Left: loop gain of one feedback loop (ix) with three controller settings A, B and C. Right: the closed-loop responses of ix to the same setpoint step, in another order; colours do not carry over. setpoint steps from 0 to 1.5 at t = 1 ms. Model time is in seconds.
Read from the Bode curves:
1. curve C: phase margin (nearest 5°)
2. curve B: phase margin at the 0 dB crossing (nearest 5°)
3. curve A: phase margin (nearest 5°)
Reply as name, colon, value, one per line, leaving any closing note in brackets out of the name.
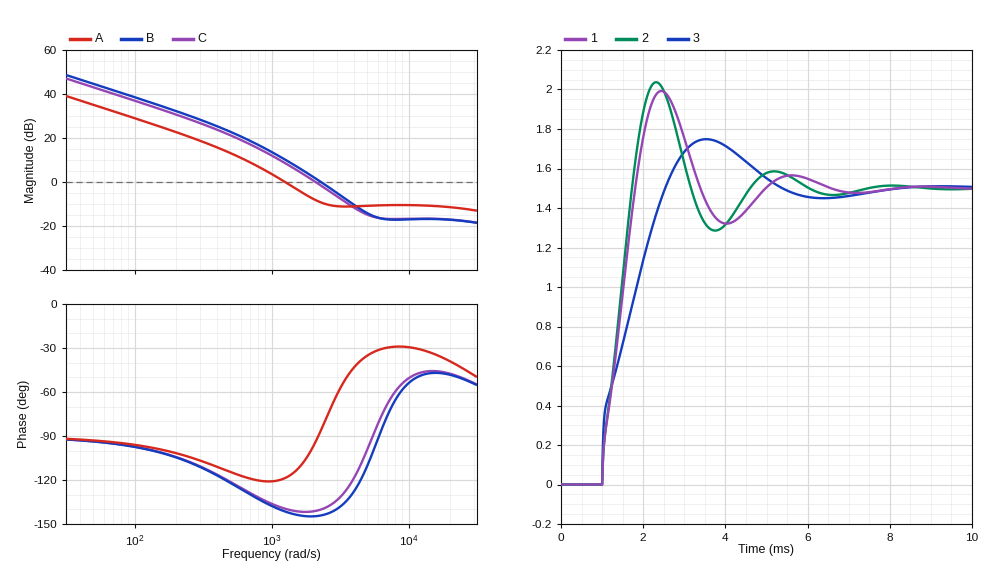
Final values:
curve C: phase margin: 40°
curve B: phase margin at the 0 dB crossing: 35°
curve A: phase margin: 60°
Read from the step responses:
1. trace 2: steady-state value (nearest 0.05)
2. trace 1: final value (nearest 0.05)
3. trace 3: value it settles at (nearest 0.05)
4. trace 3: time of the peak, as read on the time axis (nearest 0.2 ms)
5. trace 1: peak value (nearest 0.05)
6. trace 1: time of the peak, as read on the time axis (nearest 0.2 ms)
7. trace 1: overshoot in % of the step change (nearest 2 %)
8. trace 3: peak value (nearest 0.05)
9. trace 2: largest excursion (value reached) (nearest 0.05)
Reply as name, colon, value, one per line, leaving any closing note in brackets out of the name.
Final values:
trace 2: steady-state value: 1.50
trace 1: final value: 1.50
trace 3: value it settles at: 1.50
trace 3: time of the peak, as read on the time axis: 3.6 ms
trace 1: peak value: 2.00
trace 1: time of the peak, as read on the time axis: 2.4 ms
trace 1: overshoot in % of the step change: 32 %
trace 3: peak value: 1.75
trace 2: largest excursion (value reached): 2.05
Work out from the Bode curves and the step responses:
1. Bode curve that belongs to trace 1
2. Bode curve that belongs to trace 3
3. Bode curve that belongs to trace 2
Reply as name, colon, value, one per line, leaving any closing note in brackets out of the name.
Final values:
Bode curve that belongs to trace 1: C
Bode curve that belongs to trace 3: A
Bode curve that belongs to trace 2: B
